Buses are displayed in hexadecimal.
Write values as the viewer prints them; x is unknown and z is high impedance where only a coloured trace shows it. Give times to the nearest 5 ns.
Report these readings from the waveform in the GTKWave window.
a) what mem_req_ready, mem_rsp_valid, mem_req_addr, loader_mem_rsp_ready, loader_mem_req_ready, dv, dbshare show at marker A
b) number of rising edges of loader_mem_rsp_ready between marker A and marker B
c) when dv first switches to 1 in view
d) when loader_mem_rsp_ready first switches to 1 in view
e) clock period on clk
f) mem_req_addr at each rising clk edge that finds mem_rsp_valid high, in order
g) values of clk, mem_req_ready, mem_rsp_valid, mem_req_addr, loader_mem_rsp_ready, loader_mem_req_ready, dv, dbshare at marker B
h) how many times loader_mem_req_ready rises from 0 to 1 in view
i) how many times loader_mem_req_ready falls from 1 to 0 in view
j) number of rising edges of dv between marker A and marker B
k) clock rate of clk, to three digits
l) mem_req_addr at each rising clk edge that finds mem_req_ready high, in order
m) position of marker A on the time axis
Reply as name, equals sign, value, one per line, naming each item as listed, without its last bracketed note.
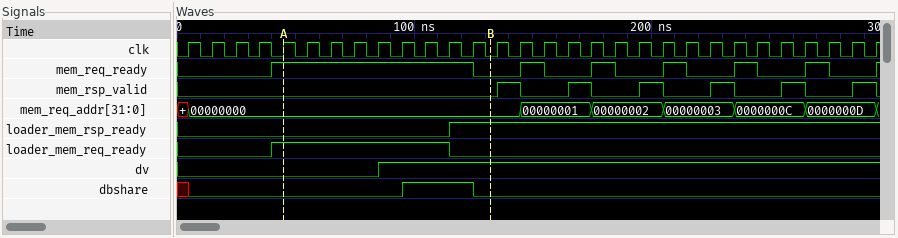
what mem_req_ready, mem_rsp_valid, mem_req_addr, loader_mem_rsp_ready, loader_mem_req_ready, dv, dbshare show at marker A = mem_req_ready=1, mem_rsp_valid=0, mem_req_addr=00000000, loader_mem_rsp_ready=0, loader_mem_req_ready=1, dv=0, dbshare=0
number of rising edges of loader_mem_rsp_ready between marker A and marker B = 1
when dv first switches to 1 in view = 85 ns
when loader_mem_rsp_ready first switches to 1 in view = 115 ns
clock period on clk = 10 ns
mem_req_addr at each rising clk edge that finds mem_rsp_valid high, in order = 00000000, 00000001, 00000002, 00000003, 0000000C, 0000000D
values of clk, mem_req_ready, mem_rsp_valid, mem_req_addr, loader_mem_rsp_ready, loader_mem_req_ready, dv, dbshare at marker B = clk=0, mem_req_ready=0, mem_rsp_valid=0, mem_req_addr=00000000, loader_mem_rsp_ready=1, loader_mem_req_ready=0, dv=1, dbshare=0
how many times loader_mem_req_ready rises from 0 to 1 in view = 1
how many times loader_mem_req_ready falls from 1 to 0 in view = 1
number of rising edges of dv between marker A and marker B = 1
clock rate of clk, to three digits = 100 MHz
mem_req_addr at each rising clk edge that finds mem_req_ready high, in order = 00000000, 00000000, 00000000, 00000000, 00000000, 00000000, 00000000, 00000000, 00000000, 00000001, 00000002, 00000003, 0000000C, 0000000D
position of marker A on the time axis = 45 ns
